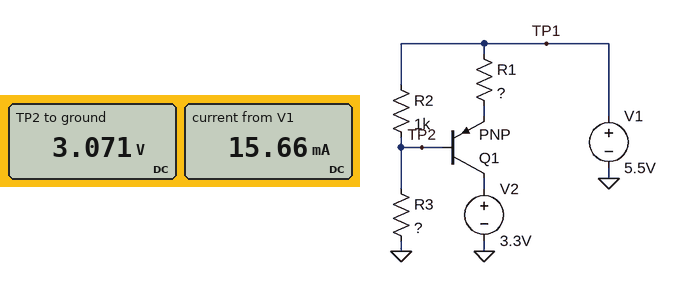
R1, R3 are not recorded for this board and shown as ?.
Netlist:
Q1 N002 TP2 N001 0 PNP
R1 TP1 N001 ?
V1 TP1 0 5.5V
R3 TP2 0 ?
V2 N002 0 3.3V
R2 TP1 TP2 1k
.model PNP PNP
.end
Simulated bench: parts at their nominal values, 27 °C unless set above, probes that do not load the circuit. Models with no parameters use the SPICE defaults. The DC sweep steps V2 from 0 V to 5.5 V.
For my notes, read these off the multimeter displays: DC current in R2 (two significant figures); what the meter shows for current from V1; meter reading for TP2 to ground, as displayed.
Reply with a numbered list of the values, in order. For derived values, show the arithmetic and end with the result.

1. (5.5 V - 3.071 V) / 1 kΩ = 2.4 mA
2. 15.66 mA
3. 3.071 V
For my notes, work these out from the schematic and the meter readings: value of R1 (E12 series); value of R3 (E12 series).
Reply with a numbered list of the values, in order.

1. 120 Ω
2. 1.2 kΩ
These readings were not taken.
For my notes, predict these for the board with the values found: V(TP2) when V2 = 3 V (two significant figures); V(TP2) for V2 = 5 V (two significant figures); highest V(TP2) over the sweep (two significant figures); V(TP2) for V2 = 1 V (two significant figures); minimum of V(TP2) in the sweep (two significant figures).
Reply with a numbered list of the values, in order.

1. 3.1 V
2. 4.2 V
3. 4.7 V
4. 3.1 V
5. 3.1 V
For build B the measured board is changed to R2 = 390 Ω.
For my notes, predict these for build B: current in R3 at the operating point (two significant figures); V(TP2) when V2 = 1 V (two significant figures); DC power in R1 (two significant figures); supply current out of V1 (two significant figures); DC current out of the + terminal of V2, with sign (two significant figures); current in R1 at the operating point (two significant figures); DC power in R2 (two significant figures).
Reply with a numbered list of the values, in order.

1. 3.5 mA
2. 4.2 V
3. 2.3 mW
4. 7.8 mA
5. -4.3 mA
6. 4.4 mA
7. 4.6 mW
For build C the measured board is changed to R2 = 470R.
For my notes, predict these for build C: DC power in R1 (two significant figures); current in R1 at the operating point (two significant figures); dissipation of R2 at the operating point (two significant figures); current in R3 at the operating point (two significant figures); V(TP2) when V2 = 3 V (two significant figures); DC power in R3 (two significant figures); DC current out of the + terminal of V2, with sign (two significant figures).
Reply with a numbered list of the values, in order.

1. 4.2 mW
2. 5.9 mA
3. 5.0 mW
4. 3.3 mA
5. 4.0 V
6. 13 mW
7. -5.8 mA
